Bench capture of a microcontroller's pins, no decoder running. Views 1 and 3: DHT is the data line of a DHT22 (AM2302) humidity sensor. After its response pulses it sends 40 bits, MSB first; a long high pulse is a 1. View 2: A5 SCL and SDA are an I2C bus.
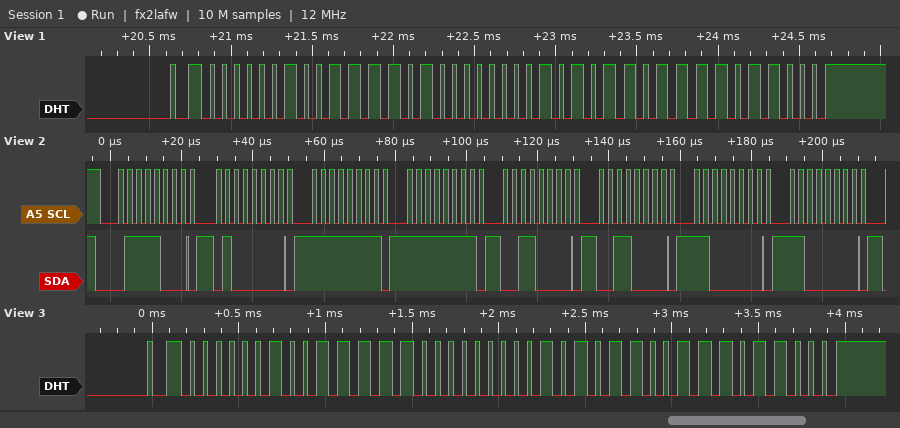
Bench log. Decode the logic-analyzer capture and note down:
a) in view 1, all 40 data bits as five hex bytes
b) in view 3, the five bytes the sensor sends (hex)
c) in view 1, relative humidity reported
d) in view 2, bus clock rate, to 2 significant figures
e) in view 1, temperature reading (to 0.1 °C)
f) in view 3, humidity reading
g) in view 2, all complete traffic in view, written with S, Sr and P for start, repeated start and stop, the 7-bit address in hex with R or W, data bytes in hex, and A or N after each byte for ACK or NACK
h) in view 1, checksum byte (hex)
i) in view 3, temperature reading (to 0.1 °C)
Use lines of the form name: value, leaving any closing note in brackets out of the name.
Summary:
in view 1, all 40 data bits as five hex bytes: 02 7A 01 5B D8
in view 3, the five bytes the sensor sends: 02 7C 01 59 D8
in view 1, relative humidity reported: 63.4 %
in view 2, bus clock rate, to 2 significant figures: 400 kHz
in view 1, temperature reading: 34.7 °C
in view 3, humidity reading: 63.6 %
in view 2, all complete traffic in view, written with S, Sr and P for start, repeated start and stop, the 7-bit address in hex with R or W, data bytes in hex, and A or N after each byte for ACK or NACK: S 3CW A 40 A FF A FF A 30 A 30 A C0 A C0 A
in view 1, checksum byte: 0xD8
in view 3, temperature reading: 34.5 °C
